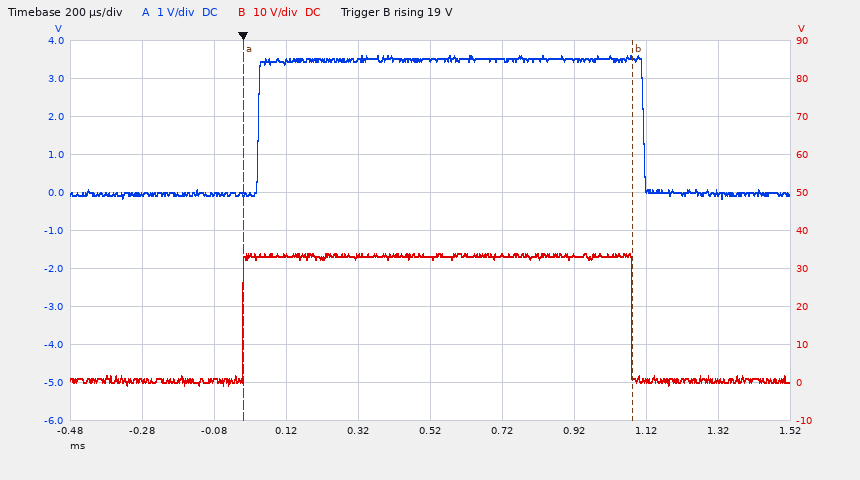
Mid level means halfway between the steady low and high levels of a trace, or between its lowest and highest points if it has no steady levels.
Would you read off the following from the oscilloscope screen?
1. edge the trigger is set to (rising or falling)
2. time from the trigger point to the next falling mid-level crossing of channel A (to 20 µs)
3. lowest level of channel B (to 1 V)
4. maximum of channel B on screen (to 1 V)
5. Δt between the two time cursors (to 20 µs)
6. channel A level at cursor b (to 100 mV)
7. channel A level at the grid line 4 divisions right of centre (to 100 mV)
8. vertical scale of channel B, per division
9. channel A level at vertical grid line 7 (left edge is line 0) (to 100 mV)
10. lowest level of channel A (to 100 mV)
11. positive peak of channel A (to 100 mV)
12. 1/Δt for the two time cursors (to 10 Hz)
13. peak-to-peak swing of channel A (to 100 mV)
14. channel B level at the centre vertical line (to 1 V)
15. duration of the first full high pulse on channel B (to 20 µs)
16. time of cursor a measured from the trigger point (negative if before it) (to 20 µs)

rising
1.12 ms
-1 V
34 V
1.08 ms
3.5 V
0.0 V
10 V
3.5 V
-200 mV
3.6 V
930 Hz
3.8 V
33 V
1.08 ms
0 µs
